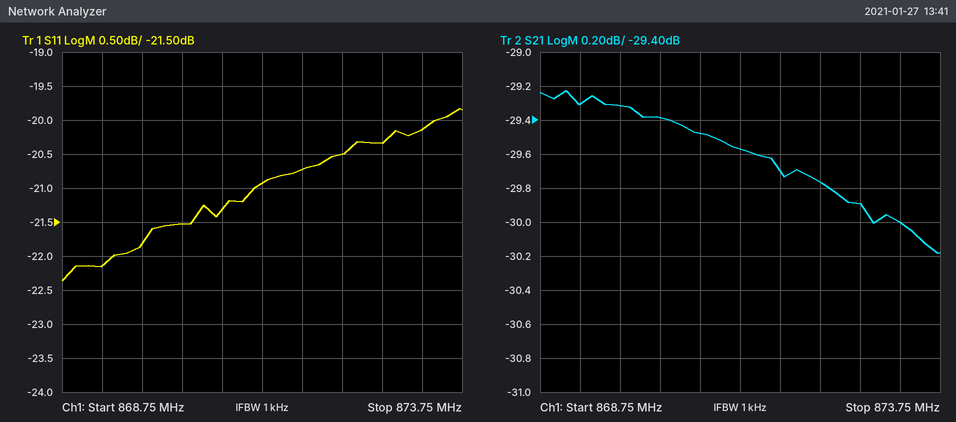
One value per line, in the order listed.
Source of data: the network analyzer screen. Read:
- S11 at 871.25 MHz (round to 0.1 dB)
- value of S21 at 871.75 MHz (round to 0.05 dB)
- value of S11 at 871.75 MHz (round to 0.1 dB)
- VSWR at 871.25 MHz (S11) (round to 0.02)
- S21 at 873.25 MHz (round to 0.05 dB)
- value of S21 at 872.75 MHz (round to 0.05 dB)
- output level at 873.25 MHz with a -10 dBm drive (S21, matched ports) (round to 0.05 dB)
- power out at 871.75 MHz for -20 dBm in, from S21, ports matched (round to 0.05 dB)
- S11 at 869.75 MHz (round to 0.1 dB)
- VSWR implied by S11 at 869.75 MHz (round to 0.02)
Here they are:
-20.9 dB
-29.70 dB
-20.7 dB
1.20
-30.00 dB
-29.90 dB
-40.00 dBm
-49.70 dBm
-21.8 dB
1.18
